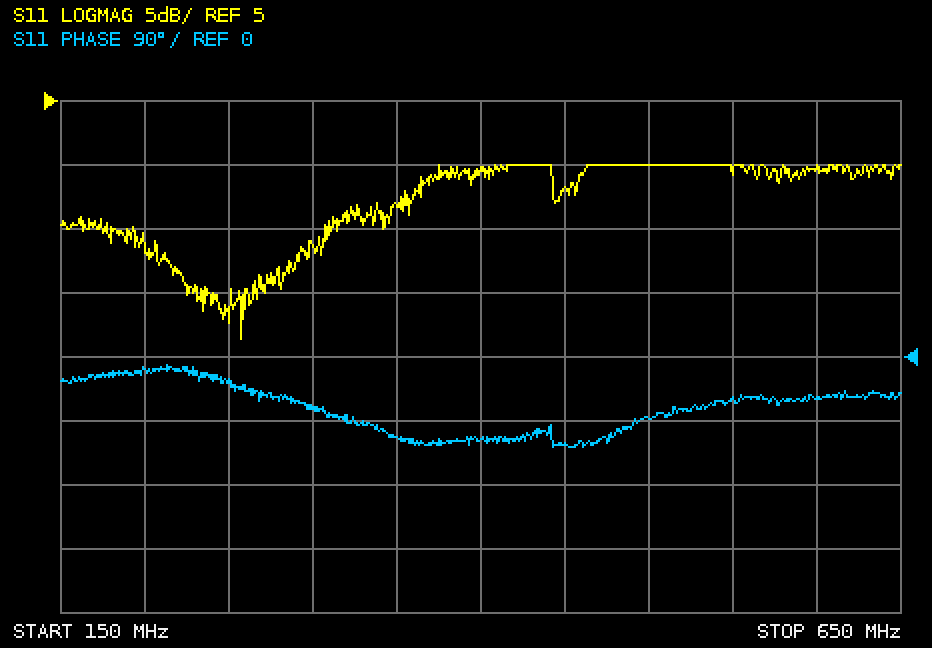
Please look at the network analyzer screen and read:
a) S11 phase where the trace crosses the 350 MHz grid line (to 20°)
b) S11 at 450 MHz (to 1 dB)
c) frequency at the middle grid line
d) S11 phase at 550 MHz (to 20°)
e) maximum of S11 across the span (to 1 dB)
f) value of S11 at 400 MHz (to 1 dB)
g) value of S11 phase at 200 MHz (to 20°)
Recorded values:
-120°
-2 dB
400 MHz
-60°
0 dB
0 dB
-20°
